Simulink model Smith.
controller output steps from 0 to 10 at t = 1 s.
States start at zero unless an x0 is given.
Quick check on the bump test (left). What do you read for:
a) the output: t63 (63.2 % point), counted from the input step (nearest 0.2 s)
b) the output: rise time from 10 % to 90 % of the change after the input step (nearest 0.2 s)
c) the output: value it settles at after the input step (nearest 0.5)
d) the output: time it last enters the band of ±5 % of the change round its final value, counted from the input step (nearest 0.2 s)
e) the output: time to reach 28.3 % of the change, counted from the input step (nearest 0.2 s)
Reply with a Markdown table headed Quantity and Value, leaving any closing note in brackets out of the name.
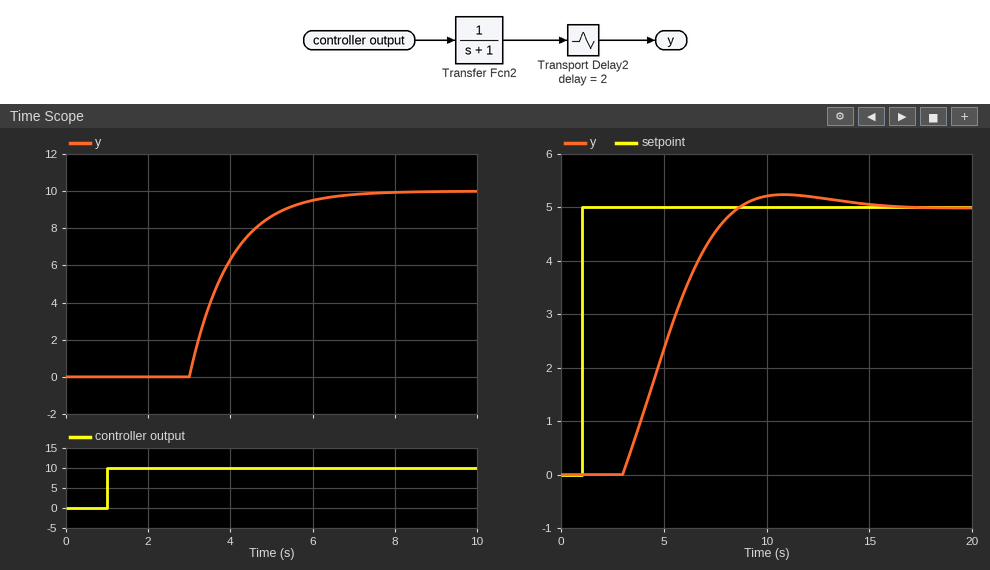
| Quantity | Value |
|---|---|
| the output: t63 (63.2 % point), counted from the input step | 3.0 s |
| the output: rise time from 10 % to 90 % of the change after the input step | 2.2 s |
| the output: value it settles at after the input step | 10.0 |
| the output: time it last enters the band of ±5 % of the change round its final value, counted from the input step | 5.0 s |
| the output: time to reach 28.3 % of the change, counted from the input step | 2.4 s |
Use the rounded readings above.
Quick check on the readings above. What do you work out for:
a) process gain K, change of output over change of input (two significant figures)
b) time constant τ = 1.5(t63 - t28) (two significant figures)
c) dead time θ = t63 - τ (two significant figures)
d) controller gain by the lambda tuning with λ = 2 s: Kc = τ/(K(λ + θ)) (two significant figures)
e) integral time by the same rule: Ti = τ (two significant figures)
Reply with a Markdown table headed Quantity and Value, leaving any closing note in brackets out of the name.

| Quantity | Value |
|---|---|
| process gain K, change of output over change of input | 1.0 |
| time constant τ = 1.5(t63 - t28) | 0.90 s |
| dead time θ = t63 - τ | 2.1 s |
| controller gain by the lambda tuning with λ = 2 s: Kc = τ/(K(λ + θ)) | 0.22 |
| integral time by the same rule: Ti = τ | 0.90 s |
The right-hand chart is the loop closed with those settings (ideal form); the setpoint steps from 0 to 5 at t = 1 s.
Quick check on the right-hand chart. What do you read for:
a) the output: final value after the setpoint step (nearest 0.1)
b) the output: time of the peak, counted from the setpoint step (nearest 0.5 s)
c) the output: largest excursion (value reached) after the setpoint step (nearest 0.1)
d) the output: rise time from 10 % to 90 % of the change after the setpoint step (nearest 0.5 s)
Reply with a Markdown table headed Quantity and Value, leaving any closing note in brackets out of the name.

| Quantity | Value |
|---|---|
| the output: final value after the setpoint step | 5.0 |
| the output: time of the peak, counted from the setpoint step | 10.0 s |
| the output: largest excursion (value reached) after the setpoint step | 5.2 |
| the output: rise time from 10 % to 90 % of the change after the setpoint step | 4.0 s |
